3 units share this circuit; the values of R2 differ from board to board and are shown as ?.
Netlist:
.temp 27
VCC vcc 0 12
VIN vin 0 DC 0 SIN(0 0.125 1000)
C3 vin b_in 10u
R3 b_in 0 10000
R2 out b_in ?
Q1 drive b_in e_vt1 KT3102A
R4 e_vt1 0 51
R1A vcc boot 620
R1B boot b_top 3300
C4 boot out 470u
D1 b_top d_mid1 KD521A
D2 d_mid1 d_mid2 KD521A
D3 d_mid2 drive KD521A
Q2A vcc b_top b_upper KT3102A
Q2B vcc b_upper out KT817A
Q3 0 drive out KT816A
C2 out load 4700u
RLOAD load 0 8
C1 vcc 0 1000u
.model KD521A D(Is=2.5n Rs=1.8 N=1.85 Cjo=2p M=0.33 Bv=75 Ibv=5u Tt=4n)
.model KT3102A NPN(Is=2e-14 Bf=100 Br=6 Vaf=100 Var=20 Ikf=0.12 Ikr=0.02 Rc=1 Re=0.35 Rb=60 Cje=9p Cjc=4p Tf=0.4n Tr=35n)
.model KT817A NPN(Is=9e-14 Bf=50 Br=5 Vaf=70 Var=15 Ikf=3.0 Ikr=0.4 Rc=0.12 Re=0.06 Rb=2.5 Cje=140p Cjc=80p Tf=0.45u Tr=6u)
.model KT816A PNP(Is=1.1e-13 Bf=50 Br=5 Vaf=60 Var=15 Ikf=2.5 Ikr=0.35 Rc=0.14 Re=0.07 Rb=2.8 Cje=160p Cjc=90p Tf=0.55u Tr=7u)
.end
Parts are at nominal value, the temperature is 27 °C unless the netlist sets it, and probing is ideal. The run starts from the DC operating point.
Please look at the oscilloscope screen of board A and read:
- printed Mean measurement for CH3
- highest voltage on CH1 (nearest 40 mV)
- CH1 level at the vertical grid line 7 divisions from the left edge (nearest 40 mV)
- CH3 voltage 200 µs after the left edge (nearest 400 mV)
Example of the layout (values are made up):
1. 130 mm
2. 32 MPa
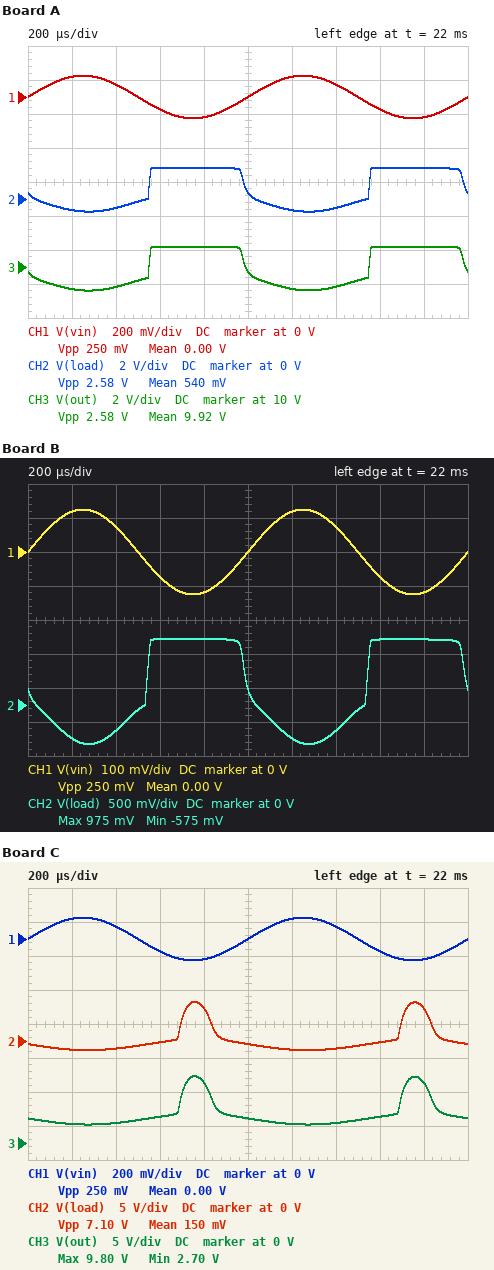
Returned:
1. 9.92 V
2. 120 mV
3. 80 mV
4. 8.8 V
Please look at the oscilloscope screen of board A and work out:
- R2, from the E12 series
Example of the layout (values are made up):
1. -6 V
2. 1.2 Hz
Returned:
1. 120 kΩ
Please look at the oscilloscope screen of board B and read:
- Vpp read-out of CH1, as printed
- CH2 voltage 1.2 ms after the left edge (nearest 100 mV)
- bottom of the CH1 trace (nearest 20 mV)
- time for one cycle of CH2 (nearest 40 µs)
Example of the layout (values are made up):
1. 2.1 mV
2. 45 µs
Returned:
1. 250 mV
2. -500 mV
3. -120 mV
4. 1.00 ms
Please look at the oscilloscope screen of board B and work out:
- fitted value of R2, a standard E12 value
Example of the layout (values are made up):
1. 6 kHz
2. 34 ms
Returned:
1. 150 kΩ
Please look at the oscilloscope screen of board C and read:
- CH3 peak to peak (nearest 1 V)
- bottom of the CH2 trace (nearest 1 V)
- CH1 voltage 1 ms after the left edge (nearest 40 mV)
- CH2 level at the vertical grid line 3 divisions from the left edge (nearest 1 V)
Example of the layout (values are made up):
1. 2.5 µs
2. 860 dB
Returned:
1. 7 V
2. -1 V
3. 0 V
4. 0 V
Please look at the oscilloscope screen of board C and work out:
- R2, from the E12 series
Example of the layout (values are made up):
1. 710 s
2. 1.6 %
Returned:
1. 27 kΩ
